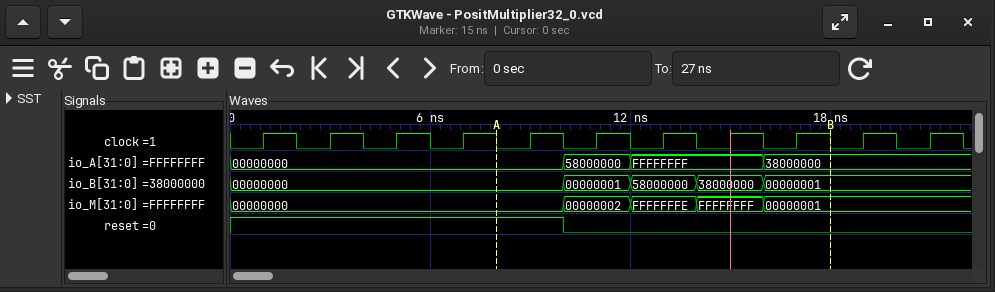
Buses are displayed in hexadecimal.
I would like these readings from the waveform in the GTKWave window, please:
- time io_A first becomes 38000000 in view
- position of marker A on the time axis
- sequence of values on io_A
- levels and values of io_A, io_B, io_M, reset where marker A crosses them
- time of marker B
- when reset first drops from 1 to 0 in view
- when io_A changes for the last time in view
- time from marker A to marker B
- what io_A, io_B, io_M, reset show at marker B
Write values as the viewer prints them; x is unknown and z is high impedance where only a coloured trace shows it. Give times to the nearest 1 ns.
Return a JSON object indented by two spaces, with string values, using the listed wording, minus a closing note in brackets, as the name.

{
  "time io_A first becomes 38000000 in view": "16 ns",
  "position of marker A on the time axis": "8 ns",
  "sequence of values on io_A": "00000000, 58000000, FFFFFFFF, 38000000",
  "levels and values of io_A, io_B, io_M, reset where marker A crosses them": "io_A=00000000, io_B=00000000, io_M=00000000, reset=1",
  "time of marker B": "18 ns",
  "when reset first drops from 1 to 0 in view": "10 ns",
  "when io_A changes for the last time in view": "16 ns",
  "time from marker A to marker B": "10 ns",
  "what io_A, io_B, io_M, reset show at marker B": "io_A=38000000, io_B=00000001, io_M=00000001, reset=0"
}
